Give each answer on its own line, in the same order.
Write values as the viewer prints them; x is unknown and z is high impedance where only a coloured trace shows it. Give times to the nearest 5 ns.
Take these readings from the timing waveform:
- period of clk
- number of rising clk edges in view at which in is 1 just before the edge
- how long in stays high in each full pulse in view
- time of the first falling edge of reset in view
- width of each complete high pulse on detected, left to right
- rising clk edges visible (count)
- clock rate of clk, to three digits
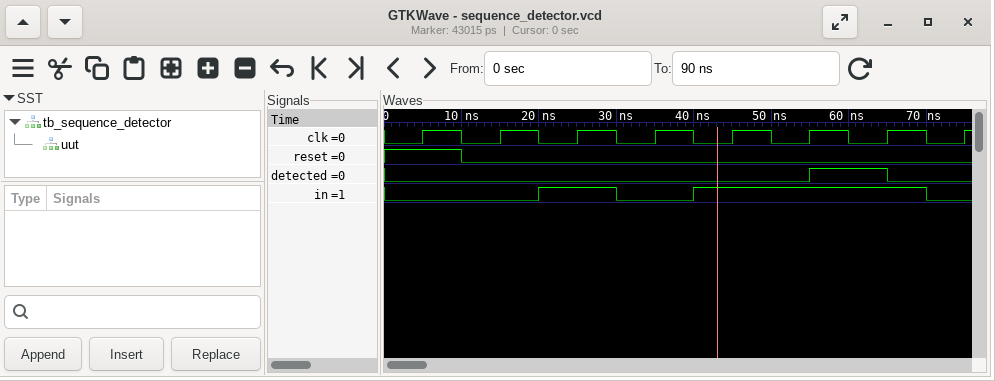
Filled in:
10 ns
4
10 ns, 30 ns
10 ns
10 ns
8
100 MHz
